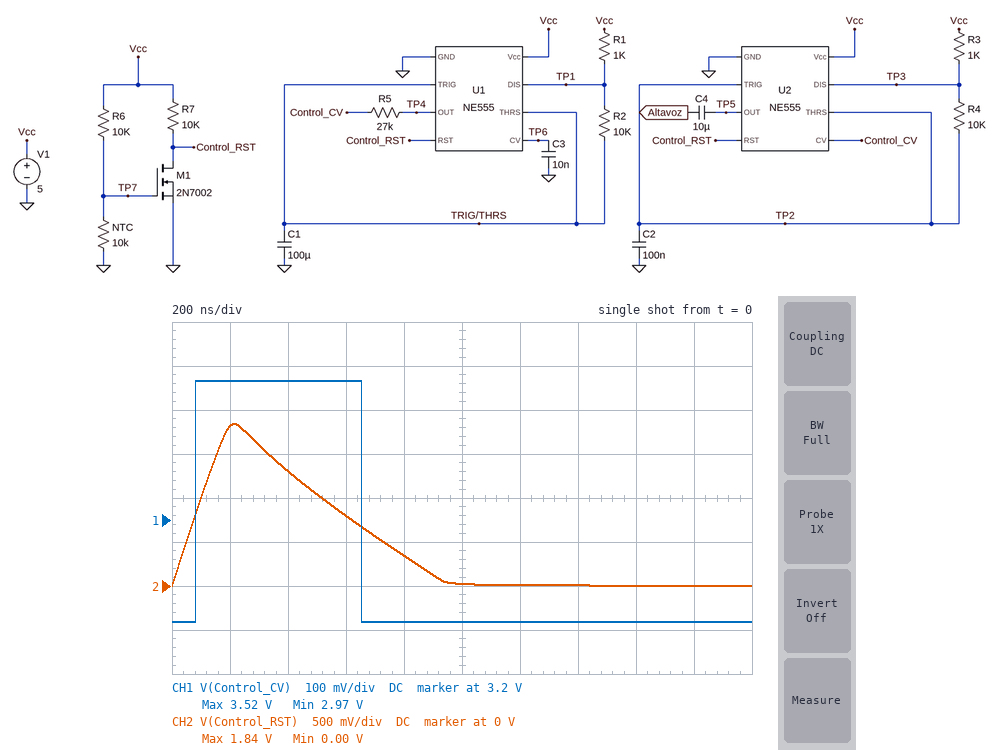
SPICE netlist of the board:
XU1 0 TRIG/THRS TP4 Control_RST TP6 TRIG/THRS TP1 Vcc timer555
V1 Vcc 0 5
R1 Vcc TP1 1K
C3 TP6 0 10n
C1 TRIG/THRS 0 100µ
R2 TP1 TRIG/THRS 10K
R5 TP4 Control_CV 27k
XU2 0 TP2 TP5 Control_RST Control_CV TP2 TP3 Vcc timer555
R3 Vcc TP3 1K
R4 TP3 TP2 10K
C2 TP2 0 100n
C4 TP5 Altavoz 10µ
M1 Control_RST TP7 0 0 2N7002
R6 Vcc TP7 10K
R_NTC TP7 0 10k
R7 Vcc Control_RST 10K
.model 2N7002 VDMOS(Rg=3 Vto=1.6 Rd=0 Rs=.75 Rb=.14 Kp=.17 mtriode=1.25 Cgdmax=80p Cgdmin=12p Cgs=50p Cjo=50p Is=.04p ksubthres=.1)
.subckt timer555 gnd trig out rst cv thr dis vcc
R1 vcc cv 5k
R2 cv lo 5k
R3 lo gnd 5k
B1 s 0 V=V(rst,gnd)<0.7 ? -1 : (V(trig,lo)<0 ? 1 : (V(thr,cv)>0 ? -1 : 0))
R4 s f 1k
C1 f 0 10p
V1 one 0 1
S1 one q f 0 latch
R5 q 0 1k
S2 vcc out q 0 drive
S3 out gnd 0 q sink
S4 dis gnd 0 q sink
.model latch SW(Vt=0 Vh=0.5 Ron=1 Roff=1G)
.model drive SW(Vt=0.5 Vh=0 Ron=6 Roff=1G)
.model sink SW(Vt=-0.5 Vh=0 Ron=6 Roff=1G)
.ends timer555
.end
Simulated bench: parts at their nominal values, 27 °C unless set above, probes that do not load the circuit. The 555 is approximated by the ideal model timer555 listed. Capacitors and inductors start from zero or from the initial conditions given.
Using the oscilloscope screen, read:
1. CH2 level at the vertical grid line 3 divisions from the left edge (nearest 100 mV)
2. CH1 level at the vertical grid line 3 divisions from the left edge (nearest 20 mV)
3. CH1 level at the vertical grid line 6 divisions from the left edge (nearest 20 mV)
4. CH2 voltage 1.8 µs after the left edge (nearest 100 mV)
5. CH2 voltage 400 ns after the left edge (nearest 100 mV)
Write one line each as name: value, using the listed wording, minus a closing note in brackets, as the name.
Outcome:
CH2 level at the vertical grid line 3 divisions from the left edge: 800 mV
CH1 level at the vertical grid line 3 divisions from the left edge: 3.52 V
CH1 level at the vertical grid line 6 divisions from the left edge: 2.96 V
CH2 voltage 1.8 µs after the left edge: 0 V
CH2 voltage 400 ns after the left edge: 1.3 V
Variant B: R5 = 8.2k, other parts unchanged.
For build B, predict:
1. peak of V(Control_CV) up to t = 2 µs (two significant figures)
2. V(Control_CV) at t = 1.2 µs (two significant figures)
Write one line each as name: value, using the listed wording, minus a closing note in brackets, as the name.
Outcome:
peak of V(Control_CV) up to t = 2 µs: 3.8 V
V(Control_CV) at t = 1.2 µs: 2.4 V
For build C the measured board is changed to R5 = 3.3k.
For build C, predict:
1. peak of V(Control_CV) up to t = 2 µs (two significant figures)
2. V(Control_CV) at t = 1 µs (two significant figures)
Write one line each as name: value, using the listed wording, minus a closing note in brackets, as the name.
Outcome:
peak of V(Control_CV) up to t = 2 µs: 4.2 V
V(Control_CV) at t = 1 µs: 1.7 V
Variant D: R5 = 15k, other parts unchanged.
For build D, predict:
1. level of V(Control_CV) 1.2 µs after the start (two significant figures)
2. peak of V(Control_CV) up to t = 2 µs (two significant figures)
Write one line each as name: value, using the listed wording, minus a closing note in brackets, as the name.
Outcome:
level of V(Control_CV) 1.2 µs after the start: 2.7 V
peak of V(Control_CV) up to t = 2 µs: 3.6 V
